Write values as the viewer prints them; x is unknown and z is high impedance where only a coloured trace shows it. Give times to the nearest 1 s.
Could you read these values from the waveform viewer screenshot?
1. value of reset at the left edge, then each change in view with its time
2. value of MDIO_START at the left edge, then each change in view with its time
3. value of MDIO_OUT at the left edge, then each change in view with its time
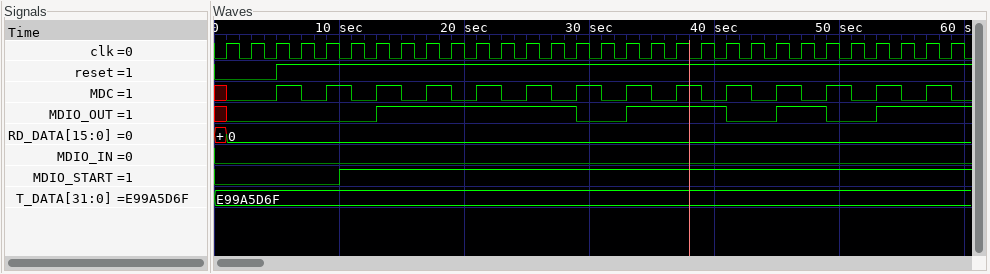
0, 1 at 5 s
0, 1 at 10 s
x, 0 at 1 s, 1 at 13 s, 0 at 29 s, 1 at 33 s, 0 at 41 s, 1 at 45 s, 0 at 49 s, 1 at 53 s
